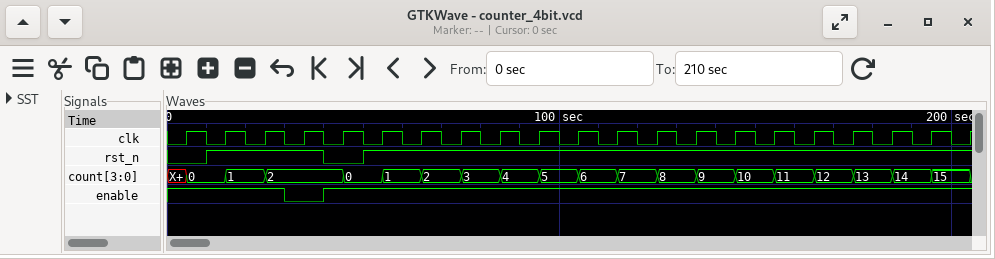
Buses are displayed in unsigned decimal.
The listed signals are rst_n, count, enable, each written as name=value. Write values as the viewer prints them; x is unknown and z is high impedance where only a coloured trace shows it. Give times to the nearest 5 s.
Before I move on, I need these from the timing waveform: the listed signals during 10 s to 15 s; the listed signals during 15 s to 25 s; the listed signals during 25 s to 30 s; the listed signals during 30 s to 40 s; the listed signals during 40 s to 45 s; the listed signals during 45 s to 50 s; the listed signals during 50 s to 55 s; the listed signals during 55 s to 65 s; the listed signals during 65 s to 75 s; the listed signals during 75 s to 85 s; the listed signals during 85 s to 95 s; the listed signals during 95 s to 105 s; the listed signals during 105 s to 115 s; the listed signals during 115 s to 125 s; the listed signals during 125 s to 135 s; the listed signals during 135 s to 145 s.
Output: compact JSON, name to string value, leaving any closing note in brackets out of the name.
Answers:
{"the listed signals during 10 s to 15 s": "rst_n=1, count=0, enable=1", "the listed signals during 15 s to 25 s": "rst_n=1, count=1, enable=1", "the listed signals during 25 s to 30 s": "rst_n=1, count=2, enable=1", "the listed signals during 30 s to 40 s": "rst_n=1, count=2, enable=0", "the listed signals during 40 s to 45 s": "rst_n=0, count=2, enable=1", "the listed signals during 45 s to 50 s": "rst_n=0, count=0, enable=1", "the listed signals during 50 s to 55 s": "rst_n=1, count=0, enable=1", "the listed signals during 55 s to 65 s": "rst_n=1, count=1, enable=1", "the listed signals during 65 s to 75 s": "rst_n=1, count=2, enable=1", "the listed signals during 75 s to 85 s": "rst_n=1, count=3, enable=1", "the listed signals during 85 s to 95 s": "rst_n=1, count=4, enable=1", "the listed signals during 95 s to 105 s": "rst_n=1, count=5, enable=1", "the listed signals during 105 s to 115 s": "rst_n=1, count=6, enable=1", "the listed signals during 115 s to 125 s": "rst_n=1, count=7, enable=1", "the listed signals during 125 s to 135 s": "rst_n=1, count=8, enable=1", "the listed signals during 135 s to 145 s": "rst_n=1, count=9, enable=1"}
